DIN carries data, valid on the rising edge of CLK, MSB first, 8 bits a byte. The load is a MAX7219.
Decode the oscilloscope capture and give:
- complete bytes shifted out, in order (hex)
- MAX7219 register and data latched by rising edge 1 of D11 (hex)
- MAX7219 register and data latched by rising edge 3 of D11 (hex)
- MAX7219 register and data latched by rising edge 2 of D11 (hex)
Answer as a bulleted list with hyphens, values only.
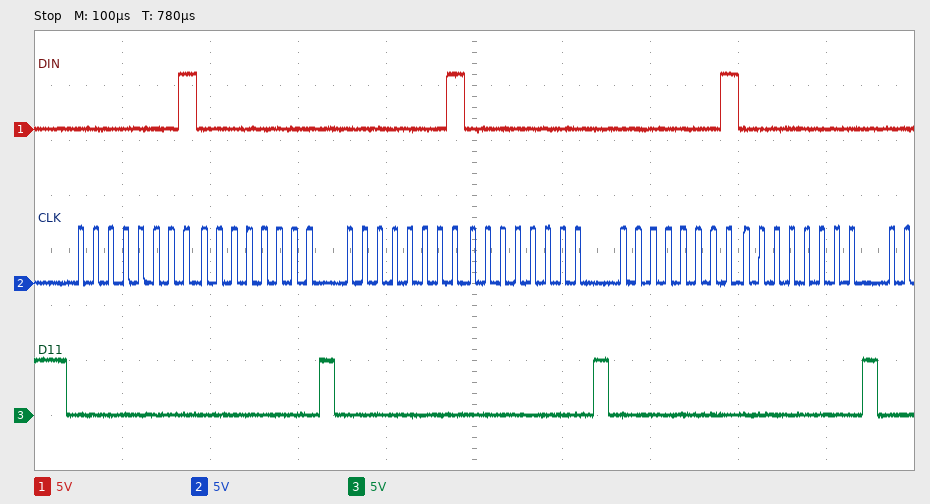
- 01 00 01 00 01 00
- register 0x1, data 0x00
- register 0x1, data 0x00
- register 0x1, data 0x00
